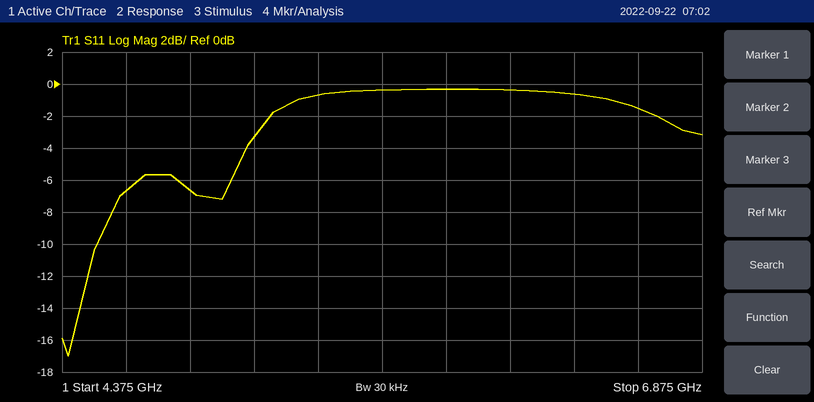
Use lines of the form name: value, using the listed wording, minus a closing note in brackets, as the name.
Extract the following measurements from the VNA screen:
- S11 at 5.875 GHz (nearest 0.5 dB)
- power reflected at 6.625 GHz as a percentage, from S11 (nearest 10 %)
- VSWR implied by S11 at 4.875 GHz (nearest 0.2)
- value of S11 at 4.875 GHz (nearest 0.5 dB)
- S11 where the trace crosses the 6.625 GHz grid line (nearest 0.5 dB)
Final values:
S11 at 5.875 GHz: -0.5 dB
power reflected at 6.625 GHz as a percentage, from S11: 70 %
VSWR implied by S11 at 4.875 GHz: 2.8
value of S11 at 4.875 GHz: -6.5 dB
S11 where the trace crosses the 6.625 GHz grid line: -1.5 dB
